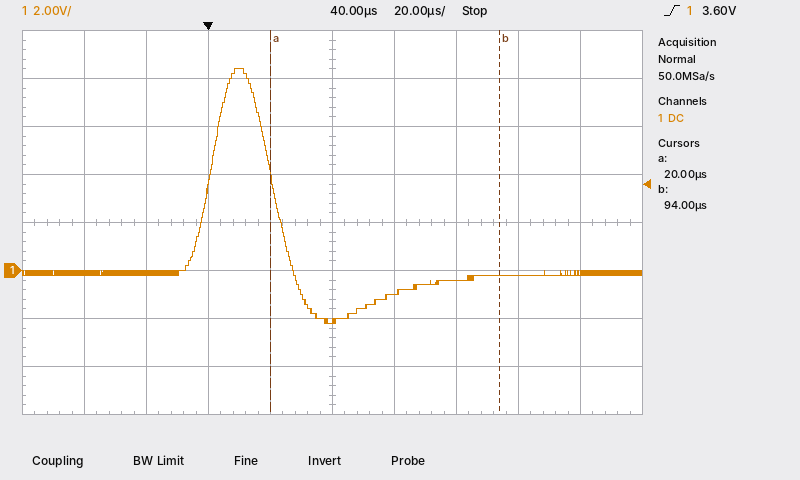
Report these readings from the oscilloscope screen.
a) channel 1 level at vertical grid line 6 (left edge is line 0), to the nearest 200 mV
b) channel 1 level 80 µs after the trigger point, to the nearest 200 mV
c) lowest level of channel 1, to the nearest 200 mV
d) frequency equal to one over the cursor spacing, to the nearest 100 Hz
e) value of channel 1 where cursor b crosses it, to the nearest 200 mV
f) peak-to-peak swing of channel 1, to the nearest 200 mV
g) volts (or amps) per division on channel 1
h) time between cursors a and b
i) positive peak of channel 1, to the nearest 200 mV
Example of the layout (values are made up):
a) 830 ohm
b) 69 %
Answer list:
a) -1.0 V
b) -400 mV
c) -2.2 V
d) 13.5 kHz
e) -200 mV
f) 10.6 V
g) 2 V
h) 74 µs
i) 8.4 V
